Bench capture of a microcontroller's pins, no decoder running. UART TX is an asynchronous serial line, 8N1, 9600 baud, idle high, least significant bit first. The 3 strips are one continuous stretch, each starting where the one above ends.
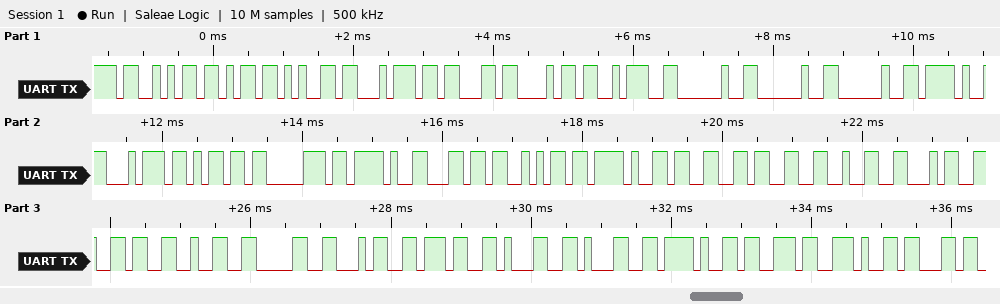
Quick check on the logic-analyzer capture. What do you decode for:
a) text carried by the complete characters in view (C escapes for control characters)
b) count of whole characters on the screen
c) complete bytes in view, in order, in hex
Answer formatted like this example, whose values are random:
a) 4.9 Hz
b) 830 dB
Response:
a) "Sketch:   /tmp/lj/33246204711/s.c"
b) 33
c) 53 6B 65 74 63 68 3A 20 20 20 2F 74 6D 70 2F 6C 6A 2F 33 33 32 34 36 32 30 34 37 31 31 2F 73 2E 63
